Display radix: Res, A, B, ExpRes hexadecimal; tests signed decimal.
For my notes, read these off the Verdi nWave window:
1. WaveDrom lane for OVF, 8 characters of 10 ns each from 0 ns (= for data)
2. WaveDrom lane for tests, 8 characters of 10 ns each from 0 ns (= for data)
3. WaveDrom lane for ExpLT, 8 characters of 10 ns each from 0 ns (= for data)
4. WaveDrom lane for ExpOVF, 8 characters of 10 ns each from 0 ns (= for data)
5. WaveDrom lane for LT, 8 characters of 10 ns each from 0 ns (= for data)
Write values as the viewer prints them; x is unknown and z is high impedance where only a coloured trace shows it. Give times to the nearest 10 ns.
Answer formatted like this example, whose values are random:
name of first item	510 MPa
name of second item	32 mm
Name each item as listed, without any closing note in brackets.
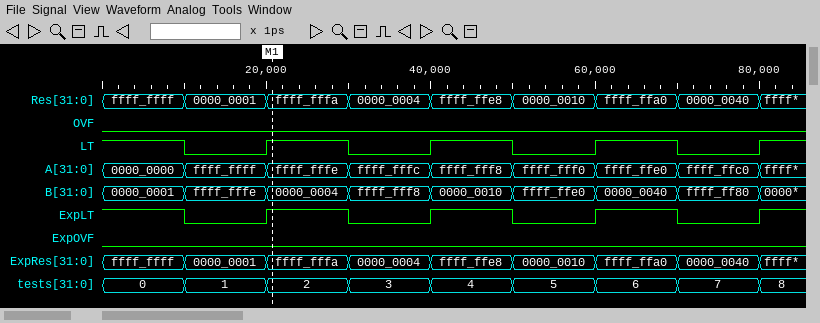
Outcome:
WaveDrom lane for OVF, 8 characters of 10 ns each from 0 ns	{name: 'OVF', wave: '0.......'}
WaveDrom lane for tests, 8 characters of 10 ns each from 0 ns	{name: 'tests', wave: '========', data: '0 1 2 3 4 5 6 7'}
WaveDrom lane for ExpLT, 8 characters of 10 ns each from 0 ns	{name: 'ExpLT', wave: '10101010'}
WaveDrom lane for ExpOVF, 8 characters of 10 ns each from 0 ns	{name: 'ExpOVF', wave: '0.......'}
WaveDrom lane for LT, 8 characters of 10 ns each from 0 ns	{name: 'LT', wave: '10101010'}
